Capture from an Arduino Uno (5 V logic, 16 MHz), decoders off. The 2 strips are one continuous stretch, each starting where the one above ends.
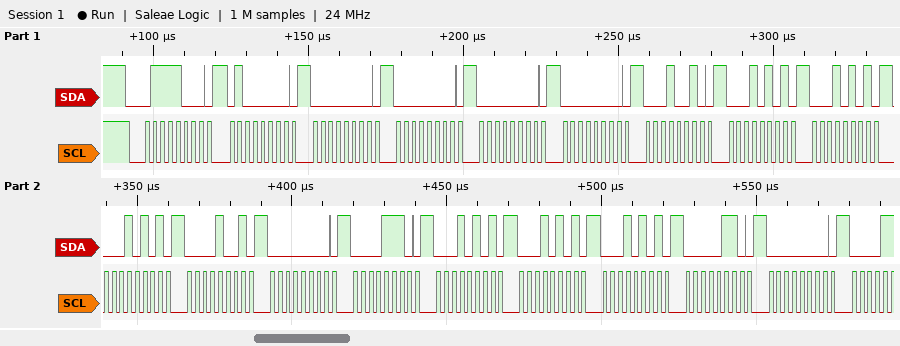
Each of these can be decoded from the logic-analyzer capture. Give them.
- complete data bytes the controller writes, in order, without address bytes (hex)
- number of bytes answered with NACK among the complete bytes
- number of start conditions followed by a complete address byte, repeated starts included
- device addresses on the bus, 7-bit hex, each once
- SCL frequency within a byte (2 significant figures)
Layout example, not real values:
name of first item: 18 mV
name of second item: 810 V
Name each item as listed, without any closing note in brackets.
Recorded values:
complete data bytes the controller writes, in order, without address bytes: 40 00 00 00 00 12 15 15 15 09 00 0E 15 15 15 06 00
number of bytes answered with NACK among the complete bytes: 0
number of start conditions followed by a complete address byte, repeated starts included: 1
device addresses on the bus, 7-bit hex, each once: 0x3C
SCL frequency within a byte: 400 kHz
